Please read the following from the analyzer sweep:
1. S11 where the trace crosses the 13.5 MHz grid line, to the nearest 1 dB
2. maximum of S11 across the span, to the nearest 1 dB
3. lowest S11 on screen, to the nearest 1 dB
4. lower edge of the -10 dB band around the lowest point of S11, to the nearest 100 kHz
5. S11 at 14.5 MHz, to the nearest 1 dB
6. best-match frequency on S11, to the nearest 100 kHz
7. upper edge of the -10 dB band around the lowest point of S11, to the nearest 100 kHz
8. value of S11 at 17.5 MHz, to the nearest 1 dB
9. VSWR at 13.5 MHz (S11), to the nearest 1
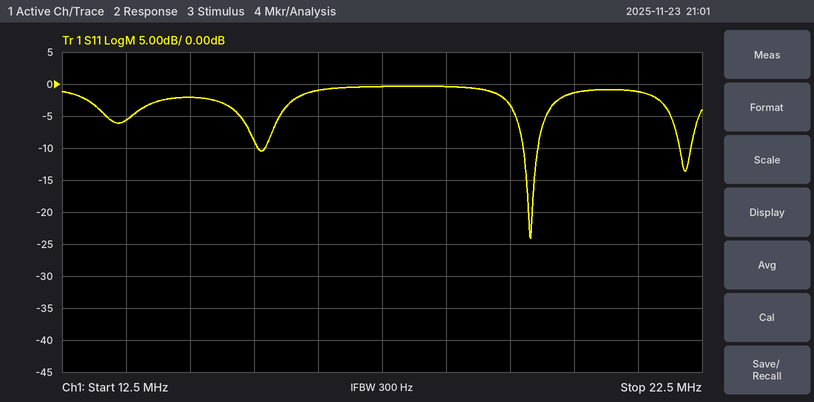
-6 dB
0 dB
-24 dB
19.7 MHz
-2 dB
19.8 MHz
19.9 MHz
0 dB
3
